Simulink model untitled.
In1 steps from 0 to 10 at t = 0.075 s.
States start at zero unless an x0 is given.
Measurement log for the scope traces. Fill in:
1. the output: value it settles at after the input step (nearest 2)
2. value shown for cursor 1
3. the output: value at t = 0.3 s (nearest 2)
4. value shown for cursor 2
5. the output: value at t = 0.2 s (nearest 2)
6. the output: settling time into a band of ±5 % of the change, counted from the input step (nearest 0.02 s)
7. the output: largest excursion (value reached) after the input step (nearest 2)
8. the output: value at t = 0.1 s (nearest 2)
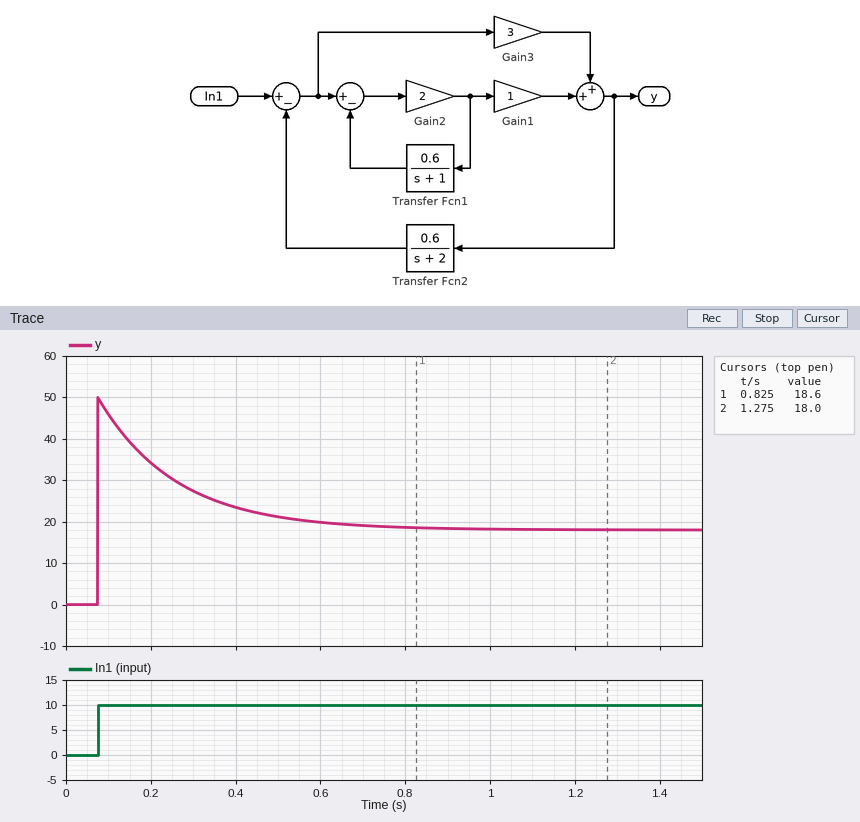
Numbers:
18
18.6
28
18.0
34
0.66 s
50
46
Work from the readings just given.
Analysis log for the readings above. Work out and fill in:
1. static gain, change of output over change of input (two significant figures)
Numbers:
1.8
